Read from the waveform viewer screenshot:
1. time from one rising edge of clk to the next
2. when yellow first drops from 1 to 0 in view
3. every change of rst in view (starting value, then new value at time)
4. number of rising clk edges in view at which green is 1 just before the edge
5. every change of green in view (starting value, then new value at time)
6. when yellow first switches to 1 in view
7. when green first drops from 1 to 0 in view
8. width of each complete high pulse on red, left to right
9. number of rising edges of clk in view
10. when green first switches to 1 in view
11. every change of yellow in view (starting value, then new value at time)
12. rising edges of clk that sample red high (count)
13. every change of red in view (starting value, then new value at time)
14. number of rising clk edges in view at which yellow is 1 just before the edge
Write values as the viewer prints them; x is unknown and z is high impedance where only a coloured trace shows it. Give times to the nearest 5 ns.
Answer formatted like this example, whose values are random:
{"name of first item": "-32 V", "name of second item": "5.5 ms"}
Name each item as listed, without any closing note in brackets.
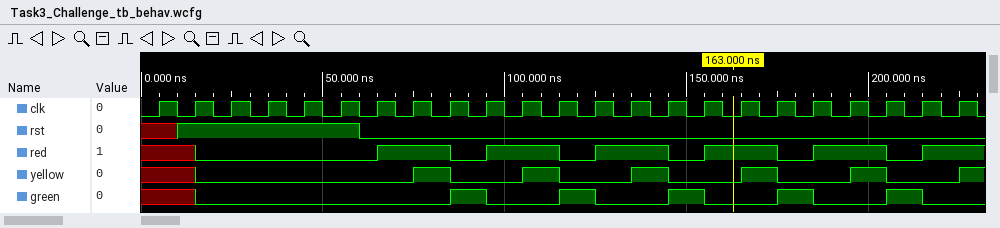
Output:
{"time from one rising edge of clk to the next": "10 ns", "when yellow first drops from 1 to 0 in view": "85 ns", "every change of rst in view": "x, 1 at 10 ns, 0 at 60 ns", "number of rising clk edges in view at which green is 1 just before the edge": "5", "every change of green in view": "x, 0 at 15 ns, 1 at 85 ns, 0 at 95 ns, 1 at 115 ns, 0 at 125 ns, 1 at 145 ns, 0 at 155 ns, 1 at 175 ns, 0 at 185 ns, 1 at 205 ns, 0 at 215 ns", "when yellow first switches to 1 in view": "75 ns", "when green first drops from 1 to 0 in view": "95 ns", "width of each complete high pulse on red, left to right": "20 ns, 20 ns, 20 ns, 20 ns, 20 ns", "number of rising edges of clk in view": "23", "when green first switches to 1 in view": "85 ns", "every change of yellow in view": "x, 0 at 15 ns, 1 at 75 ns, 0 at 85 ns, 1 at 105 ns, 0 at 115 ns, 1 at 135 ns, 0 at 145 ns, 1 at 165 ns, 0 at 175 ns, 1 at 195 ns, 0 at 205 ns, 1 at 225 ns", "rising edges of clk that sample red high": "11", "every change of red in view": "x, 0 at 15 ns, 1 at 65 ns, 0 at 85 ns, 1 at 95 ns, 0 at 115 ns, 1 at 125 ns, 0 at 145 ns, 1 at 155 ns, 0 at 175 ns, 1 at 185 ns, 0 at 205 ns, 1 at 215 ns", "number of rising clk edges in view at which yellow is 1 just before the edge": "5"}
